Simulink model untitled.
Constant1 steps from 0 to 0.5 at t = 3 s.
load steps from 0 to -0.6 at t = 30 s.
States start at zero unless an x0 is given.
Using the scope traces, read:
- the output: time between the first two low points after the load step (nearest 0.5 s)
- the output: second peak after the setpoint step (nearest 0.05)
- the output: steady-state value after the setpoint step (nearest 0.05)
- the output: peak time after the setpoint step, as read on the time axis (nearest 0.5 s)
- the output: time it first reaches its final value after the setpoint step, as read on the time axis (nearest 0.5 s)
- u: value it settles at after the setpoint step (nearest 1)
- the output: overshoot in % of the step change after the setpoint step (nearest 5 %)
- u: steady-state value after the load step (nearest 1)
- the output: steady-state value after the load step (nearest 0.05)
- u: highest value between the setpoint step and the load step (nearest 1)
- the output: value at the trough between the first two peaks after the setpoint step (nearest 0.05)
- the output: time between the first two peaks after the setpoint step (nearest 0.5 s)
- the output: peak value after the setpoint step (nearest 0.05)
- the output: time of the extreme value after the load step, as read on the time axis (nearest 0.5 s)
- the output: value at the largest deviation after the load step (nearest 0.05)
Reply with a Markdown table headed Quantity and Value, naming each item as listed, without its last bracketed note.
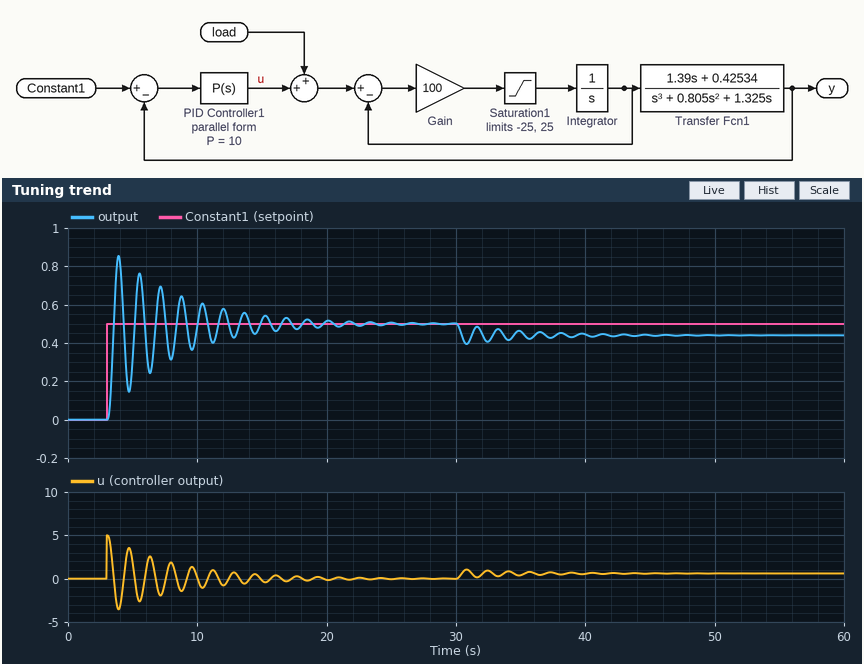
| Quantity | Value |
|---|---|
| the output: time between the first two low points after the load step | 1.5 s |
| the output: second peak after the setpoint step | 0.75 |
| the output: steady-state value after the setpoint step | 0.50 |
| the output: peak time after the setpoint step, as read on the time axis | 4.0 s |
| the output: time it first reaches its final value after the setpoint step, as read on the time axis | 3.5 s |
| u: value it settles at after the setpoint step | 0 |
| the output: overshoot in % of the step change after the setpoint step | 70 % |
| u: steady-state value after the load step | 1 |
| the output: steady-state value after the load step | 0.45 |
| u: highest value between the setpoint step and the load step | 5 |
| the output: value at the trough between the first two peaks after the setpoint step | 0.15 |
| the output: time between the first two peaks after the setpoint step | 1.5 s |
| the output: peak value after the setpoint step | 0.85 |
| the output: time of the extreme value after the load step, as read on the time axis | 31.0 s |
| the output: value at the largest deviation after the load step | 0.40 |
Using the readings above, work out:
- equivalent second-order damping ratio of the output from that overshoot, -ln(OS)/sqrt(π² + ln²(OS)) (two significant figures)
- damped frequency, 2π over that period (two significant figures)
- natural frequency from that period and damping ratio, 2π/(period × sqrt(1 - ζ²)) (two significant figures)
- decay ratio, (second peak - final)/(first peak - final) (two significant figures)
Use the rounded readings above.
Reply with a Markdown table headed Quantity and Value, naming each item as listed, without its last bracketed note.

| Quantity | Value |
|---|---|
| equivalent second-order damping ratio of the output from that overshoot, -ln(OS)/sqrt(π² + ln²(OS)) | 0.11 |
| damped frequency, 2π over that period | 4.2 rad/s |
| natural frequency from that period and damping ratio, 2π/(period × sqrt(1 - ζ²)) | 4.2 rad/s |
| decay ratio, (second peak - final)/(first peak - final) | 0.71 |
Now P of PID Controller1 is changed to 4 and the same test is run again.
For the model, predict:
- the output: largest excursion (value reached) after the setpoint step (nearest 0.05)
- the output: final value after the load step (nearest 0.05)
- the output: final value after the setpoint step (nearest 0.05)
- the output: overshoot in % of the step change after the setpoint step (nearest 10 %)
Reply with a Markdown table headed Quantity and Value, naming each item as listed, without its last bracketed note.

| Quantity | Value |
|---|---|
| the output: largest excursion (value reached) after the setpoint step | 0.75 |
| the output: final value after the load step | 0.35 |
| the output: final value after the setpoint step | 0.50 |
| the output: overshoot in % of the step change after the setpoint step | 50 % |
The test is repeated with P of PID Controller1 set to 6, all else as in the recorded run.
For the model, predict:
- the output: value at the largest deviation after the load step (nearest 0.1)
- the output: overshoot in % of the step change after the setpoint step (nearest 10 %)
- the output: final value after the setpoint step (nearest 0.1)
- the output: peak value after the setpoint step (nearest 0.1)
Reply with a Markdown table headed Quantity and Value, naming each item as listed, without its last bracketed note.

| Quantity | Value |
|---|---|
| the output: value at the largest deviation after the load step | 0.3 |
| the output: overshoot in % of the step change after the setpoint step | 60 % |
| the output: final value after the setpoint step | 0.5 |
| the output: peak value after the setpoint step | 0.8 |
